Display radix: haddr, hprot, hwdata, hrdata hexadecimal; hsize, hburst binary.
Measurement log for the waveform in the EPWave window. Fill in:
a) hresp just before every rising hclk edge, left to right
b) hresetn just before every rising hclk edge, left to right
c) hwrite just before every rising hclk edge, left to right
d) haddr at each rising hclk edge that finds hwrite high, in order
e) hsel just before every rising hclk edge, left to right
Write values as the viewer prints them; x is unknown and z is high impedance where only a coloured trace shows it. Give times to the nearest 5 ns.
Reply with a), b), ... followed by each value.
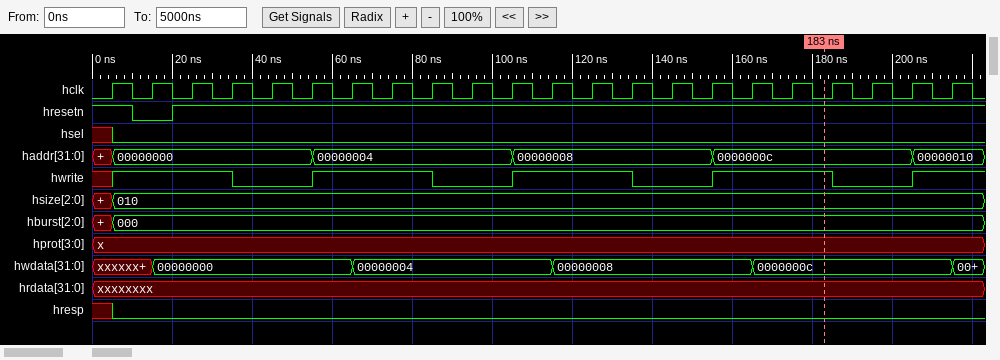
a) x 0 0 0 0 0 0 0 0 0 0 0 0 0 0 0 0 0 0 0 0 0
b) 1 0 1 1 1 1 1 1 1 1 1 1 1 1 1 1 1 1 1 1 1 1
c) x 1 1 1 0 0 1 1 1 0 0 1 1 1 0 0 1 1 1 0 0 1
d) 00000000, 00000000, 00000000, 00000004, 00000004, 00000004, 00000008, 00000008, 00000008, 0000000c, 0000000c, 0000000c, 00000010
e) x 0 0 0 0 0 0 0 0 0 0 0 0 0 0 0 0 0 0 0 0 0
